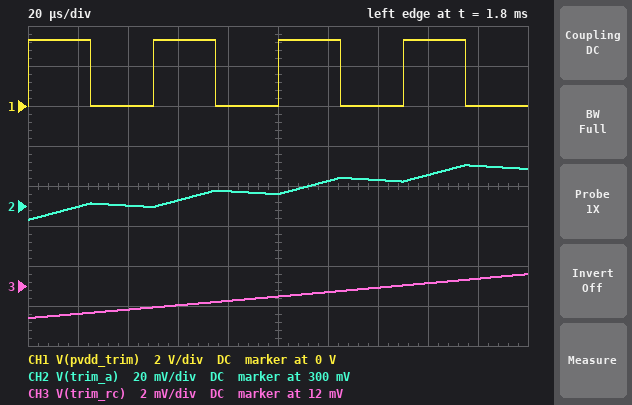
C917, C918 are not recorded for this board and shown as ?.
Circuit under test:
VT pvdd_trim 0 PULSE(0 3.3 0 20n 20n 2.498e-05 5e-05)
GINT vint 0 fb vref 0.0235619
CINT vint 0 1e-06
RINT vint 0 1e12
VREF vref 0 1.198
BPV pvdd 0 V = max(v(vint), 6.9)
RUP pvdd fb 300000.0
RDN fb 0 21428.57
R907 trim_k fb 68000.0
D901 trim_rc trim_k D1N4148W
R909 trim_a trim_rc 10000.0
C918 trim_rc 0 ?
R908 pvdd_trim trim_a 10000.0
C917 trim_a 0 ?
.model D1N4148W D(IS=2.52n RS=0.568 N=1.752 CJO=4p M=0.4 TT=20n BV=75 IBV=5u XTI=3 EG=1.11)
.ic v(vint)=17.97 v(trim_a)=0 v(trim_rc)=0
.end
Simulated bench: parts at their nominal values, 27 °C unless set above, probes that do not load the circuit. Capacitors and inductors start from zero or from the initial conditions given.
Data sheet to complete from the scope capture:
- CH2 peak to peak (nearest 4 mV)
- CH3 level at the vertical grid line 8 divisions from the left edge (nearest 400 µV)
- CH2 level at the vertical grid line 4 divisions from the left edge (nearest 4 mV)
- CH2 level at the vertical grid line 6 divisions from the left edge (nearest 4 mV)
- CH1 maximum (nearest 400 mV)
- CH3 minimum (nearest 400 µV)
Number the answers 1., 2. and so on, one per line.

1. 28 mV
2. 12.0 mV
3. 308 mV
4. 312 mV
5. 3.2 V
6. 10.4 mV
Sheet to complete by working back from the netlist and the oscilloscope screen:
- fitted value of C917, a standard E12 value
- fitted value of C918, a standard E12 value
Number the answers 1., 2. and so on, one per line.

1. 820 nF
2. 2.7 µF
